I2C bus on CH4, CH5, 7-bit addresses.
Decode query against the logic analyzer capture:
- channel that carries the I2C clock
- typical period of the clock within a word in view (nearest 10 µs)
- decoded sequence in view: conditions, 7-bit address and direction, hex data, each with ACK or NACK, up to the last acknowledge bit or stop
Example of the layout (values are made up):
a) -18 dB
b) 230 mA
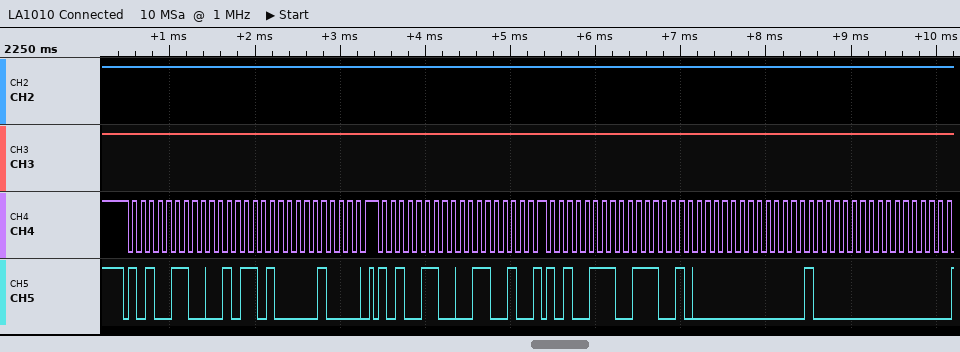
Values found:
a) CH4
b) 100 µs
c) start, address 53 write ACK, 2D ACK, 08 ACK, stop, start, address 53 write ACK, 32 ACK, repeated start, address 53 read ACK, 72 ACK, 00 ACK, 10 ACK, 00 ACK
